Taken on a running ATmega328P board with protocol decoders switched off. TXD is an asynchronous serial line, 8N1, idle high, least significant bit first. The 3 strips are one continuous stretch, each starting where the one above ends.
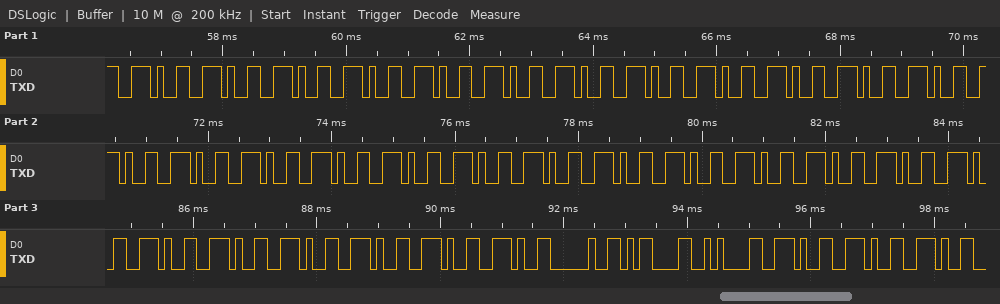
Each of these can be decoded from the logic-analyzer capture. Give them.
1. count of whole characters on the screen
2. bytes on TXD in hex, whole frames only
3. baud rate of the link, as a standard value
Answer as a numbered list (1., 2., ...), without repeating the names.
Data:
1. 37
2. 2E 2E 2E 2E 2E 2E 2E 2E 2E 2E 2E 2E 2E 2E 2E 2E 2E 2E 2E 2E 2E 2E 2E 2E 2E 2E 2E 2E 2E 2E 2E 20 0D 0A 2E 2E 2E
3. 9600 baud
